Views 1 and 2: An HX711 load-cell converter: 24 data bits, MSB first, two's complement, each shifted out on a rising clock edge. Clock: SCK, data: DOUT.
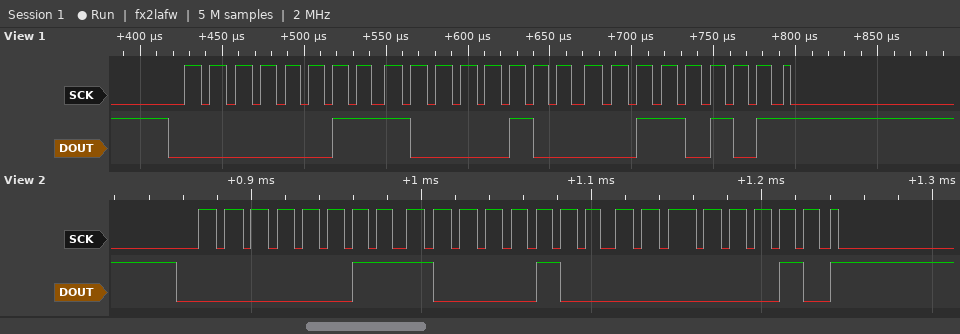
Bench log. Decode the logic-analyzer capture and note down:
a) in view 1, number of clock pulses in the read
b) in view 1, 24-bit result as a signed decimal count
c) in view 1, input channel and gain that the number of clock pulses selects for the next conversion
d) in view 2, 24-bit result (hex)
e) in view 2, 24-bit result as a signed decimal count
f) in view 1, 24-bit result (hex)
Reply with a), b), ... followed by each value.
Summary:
a) 25
b) 230453
c) channel A, gain 128
d) 0x038402
e) 230402
f) 0x038435
